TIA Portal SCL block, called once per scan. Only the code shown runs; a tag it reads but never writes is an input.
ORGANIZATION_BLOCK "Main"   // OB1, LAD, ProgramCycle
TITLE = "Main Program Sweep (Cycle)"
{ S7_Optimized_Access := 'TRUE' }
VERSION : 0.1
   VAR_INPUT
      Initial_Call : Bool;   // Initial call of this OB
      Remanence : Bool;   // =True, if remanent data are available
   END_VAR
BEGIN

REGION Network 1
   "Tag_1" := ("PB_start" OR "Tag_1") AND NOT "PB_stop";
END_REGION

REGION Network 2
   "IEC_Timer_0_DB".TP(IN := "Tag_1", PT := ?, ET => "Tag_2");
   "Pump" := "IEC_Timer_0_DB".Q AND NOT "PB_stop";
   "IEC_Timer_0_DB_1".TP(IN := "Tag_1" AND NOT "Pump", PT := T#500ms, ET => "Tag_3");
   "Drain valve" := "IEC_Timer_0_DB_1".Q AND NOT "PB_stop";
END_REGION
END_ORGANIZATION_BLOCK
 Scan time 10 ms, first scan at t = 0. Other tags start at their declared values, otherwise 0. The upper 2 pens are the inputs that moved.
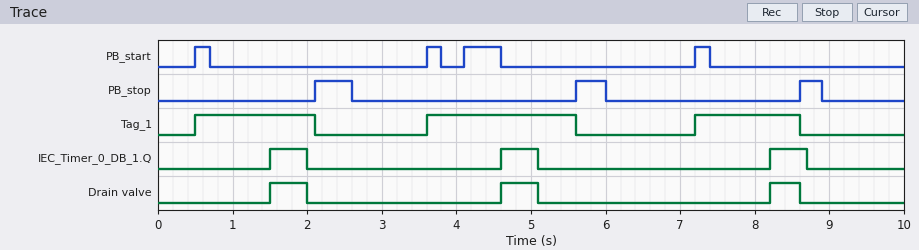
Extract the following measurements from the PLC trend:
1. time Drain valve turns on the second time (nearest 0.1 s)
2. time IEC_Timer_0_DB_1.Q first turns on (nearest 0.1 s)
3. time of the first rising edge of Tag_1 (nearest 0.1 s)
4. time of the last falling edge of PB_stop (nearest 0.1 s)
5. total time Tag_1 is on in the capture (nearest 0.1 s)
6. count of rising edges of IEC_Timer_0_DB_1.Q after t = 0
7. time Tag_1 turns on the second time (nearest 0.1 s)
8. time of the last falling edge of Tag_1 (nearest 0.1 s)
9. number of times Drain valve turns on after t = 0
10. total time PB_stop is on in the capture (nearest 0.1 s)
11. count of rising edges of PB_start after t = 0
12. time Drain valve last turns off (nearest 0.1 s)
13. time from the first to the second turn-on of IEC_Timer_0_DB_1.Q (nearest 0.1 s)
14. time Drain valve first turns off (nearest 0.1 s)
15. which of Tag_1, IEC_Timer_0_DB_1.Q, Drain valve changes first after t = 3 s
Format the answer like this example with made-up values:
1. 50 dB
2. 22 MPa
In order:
1. 4.6 s
2. 1.5 s
3. 0.5 s
4. 8.9 s
5. 5.0 s
6. 3
7. 3.6 s
8. 8.6 s
9. 3
10. 1.2 s
11. 4
12. 8.6 s
13. 3.1 s
14. 2.0 s
15. Tag_1
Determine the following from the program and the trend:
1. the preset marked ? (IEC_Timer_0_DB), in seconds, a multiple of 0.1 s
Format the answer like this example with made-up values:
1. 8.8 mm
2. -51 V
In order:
1. 1.0 s
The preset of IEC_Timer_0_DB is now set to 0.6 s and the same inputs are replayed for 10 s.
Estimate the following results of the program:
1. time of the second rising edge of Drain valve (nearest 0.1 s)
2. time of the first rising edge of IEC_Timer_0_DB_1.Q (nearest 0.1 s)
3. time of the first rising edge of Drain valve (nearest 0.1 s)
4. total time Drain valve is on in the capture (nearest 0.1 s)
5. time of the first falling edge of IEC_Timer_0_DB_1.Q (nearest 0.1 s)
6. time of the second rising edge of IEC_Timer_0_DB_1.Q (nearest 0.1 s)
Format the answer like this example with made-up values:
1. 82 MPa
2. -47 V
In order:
1. 4.2 s
2. 1.1 s
3. 1.1 s
4. 1.5 s
5. 1.6 s
6. 4.2 s
